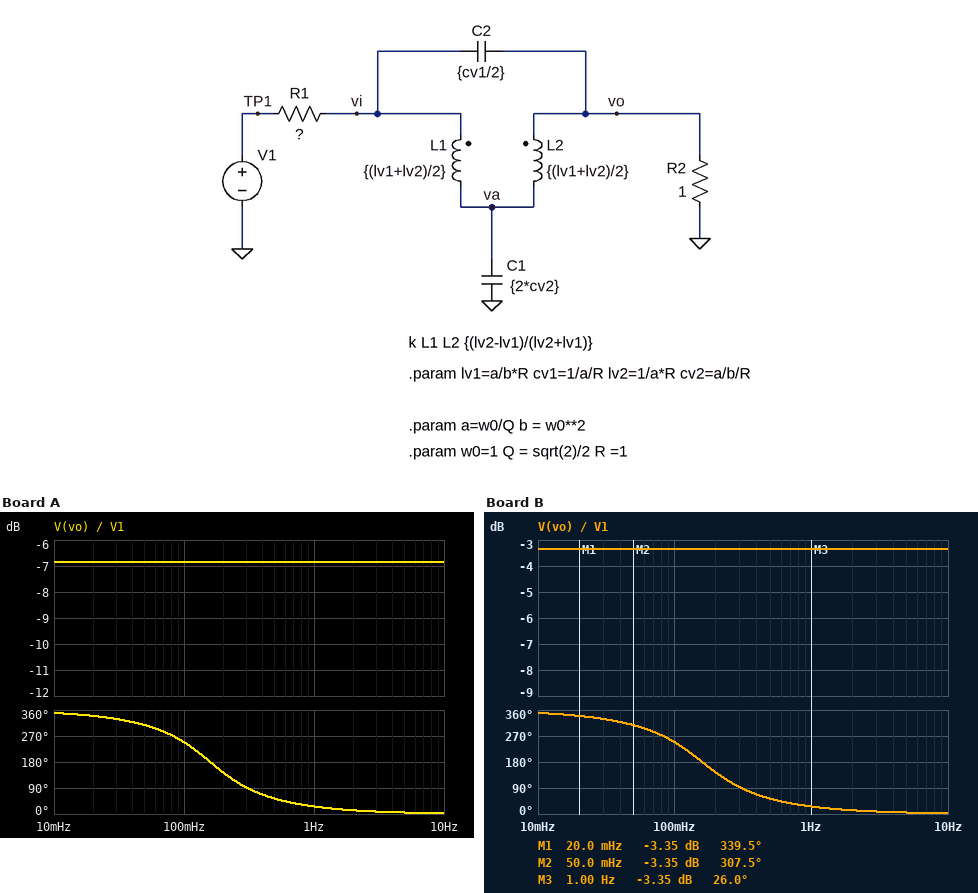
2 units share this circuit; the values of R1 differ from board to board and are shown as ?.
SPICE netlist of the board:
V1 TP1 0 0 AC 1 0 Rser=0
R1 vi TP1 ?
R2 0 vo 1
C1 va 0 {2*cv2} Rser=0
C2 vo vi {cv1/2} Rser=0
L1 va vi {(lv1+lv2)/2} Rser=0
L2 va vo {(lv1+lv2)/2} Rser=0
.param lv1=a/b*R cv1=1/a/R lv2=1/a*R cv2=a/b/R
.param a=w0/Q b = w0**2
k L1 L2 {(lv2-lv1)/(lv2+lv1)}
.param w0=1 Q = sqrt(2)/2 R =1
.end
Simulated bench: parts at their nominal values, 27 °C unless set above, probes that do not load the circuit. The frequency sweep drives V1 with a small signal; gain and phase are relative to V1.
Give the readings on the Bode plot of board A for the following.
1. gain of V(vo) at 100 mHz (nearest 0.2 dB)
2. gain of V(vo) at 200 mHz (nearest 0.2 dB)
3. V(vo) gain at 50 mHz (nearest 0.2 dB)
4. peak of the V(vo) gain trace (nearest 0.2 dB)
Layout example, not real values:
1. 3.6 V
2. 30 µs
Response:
1. -6.8 dB
2. -6.8 dB
3. -6.8 dB
4. -6.8 dB
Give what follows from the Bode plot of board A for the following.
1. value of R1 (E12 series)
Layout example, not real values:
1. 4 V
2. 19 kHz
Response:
1. 1.2 Ω
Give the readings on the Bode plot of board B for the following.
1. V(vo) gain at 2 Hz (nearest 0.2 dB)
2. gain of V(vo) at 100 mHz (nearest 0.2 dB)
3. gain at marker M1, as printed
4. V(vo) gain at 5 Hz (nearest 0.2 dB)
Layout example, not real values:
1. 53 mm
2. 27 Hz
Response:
1. -3.4 dB
2. -3.4 dB
3. -3.35 dB
4. -3.4 dB
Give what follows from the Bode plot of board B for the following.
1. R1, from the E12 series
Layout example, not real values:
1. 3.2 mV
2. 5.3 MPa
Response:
1. 0.47 Ω
